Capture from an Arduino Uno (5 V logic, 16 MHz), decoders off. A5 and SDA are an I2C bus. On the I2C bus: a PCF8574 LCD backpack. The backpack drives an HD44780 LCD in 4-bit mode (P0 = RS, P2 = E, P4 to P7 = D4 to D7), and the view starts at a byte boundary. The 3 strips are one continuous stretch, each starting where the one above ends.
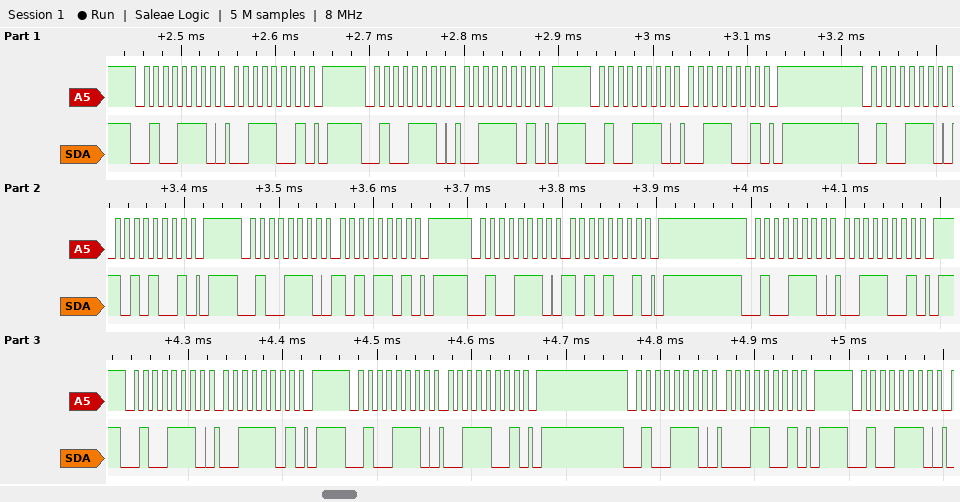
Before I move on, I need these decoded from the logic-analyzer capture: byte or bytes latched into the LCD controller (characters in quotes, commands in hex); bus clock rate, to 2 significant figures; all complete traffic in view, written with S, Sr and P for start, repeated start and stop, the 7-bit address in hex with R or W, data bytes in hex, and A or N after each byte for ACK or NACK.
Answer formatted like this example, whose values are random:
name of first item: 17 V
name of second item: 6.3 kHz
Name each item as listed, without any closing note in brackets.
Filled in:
byte or bytes latched into the LCD controller: ':'
bus clock rate, to 2 significant figures: 100 kHz
all complete traffic in view, written with S, Sr and P for start, repeated start and stop, the 7-bit address in hex with R or W, data bytes in hex, and A or N after each byte for ACK or NACK: S 27W A 39 A P S 27W A 3D A P S 27W A 39 A P S 27W A A9 A P S 27W A AD A P S 27W A A9 A P S 27W A 39 A P S 27W A 3D A P S 27W A 39 A P S 27W A 19 A P S 27W A
